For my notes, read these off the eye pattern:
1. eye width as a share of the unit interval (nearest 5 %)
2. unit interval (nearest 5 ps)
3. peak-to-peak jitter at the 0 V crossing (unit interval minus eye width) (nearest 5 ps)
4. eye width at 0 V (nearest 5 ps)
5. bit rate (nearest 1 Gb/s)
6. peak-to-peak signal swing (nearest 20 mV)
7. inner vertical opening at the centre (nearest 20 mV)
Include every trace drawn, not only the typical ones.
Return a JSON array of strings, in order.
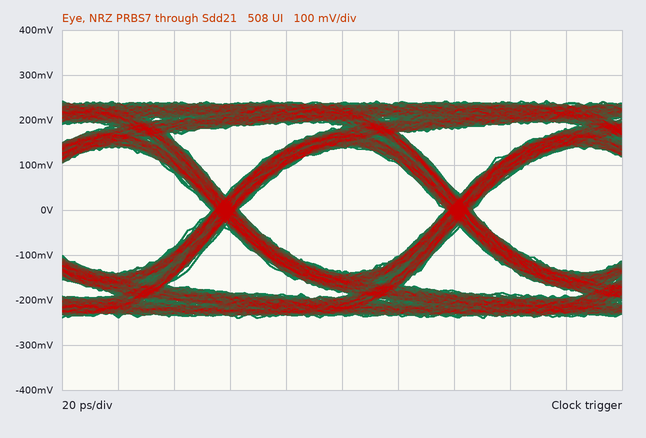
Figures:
["90 %", "85 ps", "10 ps", "75 ps", "12 Gb/s", "480 mV", "280 mV"]
